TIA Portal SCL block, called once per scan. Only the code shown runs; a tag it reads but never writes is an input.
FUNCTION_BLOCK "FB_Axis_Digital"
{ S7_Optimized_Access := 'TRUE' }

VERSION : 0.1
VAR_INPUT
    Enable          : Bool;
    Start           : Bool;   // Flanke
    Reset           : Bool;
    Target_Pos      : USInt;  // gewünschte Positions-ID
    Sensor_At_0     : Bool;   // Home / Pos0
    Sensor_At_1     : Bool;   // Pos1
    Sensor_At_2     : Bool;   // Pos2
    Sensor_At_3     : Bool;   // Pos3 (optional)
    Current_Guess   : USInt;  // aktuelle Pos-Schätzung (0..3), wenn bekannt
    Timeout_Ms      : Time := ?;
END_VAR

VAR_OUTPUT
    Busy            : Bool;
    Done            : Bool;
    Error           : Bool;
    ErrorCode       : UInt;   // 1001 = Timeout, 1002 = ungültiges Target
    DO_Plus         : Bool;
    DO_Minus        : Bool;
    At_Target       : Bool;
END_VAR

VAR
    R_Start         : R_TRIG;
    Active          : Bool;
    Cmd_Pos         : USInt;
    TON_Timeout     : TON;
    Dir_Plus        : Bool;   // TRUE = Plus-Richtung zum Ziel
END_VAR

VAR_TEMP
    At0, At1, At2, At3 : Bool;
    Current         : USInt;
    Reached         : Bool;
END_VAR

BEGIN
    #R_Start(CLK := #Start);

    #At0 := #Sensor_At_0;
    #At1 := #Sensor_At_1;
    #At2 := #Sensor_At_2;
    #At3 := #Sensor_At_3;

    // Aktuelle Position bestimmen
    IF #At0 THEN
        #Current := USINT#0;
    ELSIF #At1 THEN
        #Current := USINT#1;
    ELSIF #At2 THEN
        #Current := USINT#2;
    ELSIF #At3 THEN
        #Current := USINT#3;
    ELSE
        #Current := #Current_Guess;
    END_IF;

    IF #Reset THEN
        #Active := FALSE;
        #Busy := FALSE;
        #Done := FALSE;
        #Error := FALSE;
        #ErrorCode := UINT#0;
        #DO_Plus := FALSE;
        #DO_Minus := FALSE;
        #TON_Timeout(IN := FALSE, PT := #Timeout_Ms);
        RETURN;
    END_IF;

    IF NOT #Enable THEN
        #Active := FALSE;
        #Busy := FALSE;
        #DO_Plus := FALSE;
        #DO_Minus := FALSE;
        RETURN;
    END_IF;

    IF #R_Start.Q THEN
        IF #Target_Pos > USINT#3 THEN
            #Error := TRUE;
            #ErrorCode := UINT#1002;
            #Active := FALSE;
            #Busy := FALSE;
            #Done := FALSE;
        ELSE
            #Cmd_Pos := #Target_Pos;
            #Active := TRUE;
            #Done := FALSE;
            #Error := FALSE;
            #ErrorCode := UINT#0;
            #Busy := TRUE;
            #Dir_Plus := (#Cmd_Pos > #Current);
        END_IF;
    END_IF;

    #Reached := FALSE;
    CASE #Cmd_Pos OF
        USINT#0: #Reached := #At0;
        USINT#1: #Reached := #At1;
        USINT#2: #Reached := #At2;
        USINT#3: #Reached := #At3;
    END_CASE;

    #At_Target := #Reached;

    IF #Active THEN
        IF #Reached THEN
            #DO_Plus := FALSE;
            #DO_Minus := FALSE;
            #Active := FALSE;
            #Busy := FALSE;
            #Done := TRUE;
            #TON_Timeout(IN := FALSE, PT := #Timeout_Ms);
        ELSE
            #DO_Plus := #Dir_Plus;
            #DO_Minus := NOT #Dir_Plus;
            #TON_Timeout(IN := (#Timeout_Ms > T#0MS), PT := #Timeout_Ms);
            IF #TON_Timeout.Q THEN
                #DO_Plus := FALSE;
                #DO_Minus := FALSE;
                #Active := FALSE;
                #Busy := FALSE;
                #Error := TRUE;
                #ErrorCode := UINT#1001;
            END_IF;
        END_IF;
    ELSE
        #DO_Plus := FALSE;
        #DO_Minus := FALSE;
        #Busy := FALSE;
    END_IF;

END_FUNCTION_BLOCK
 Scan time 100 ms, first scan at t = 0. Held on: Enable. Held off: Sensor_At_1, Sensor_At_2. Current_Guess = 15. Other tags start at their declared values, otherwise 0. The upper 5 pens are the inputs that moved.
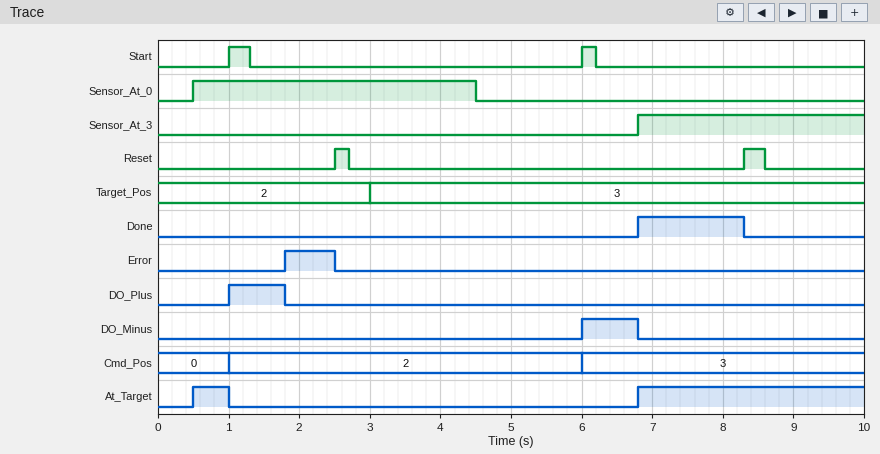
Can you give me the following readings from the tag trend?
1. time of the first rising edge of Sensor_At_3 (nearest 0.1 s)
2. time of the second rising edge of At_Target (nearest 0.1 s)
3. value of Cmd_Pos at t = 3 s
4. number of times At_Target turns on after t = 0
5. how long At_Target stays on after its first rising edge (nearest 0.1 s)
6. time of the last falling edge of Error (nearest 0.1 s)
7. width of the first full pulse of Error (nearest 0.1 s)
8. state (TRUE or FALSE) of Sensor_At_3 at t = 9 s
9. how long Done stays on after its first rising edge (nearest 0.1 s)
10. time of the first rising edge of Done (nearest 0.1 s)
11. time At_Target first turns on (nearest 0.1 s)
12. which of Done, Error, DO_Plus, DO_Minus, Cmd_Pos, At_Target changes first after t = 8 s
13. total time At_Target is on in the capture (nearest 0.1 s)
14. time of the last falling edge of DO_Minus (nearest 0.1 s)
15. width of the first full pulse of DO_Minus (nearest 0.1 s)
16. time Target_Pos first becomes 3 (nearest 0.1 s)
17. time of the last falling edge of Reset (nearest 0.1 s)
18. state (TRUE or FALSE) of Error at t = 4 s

6.8 s
6.8 s
2
2
0.5 s
2.5 s
0.7 s
TRUE
1.5 s
6.8 s
0.5 s
Done
3.7 s
6.8 s
0.8 s
3.0 s
8.6 s
FALSE
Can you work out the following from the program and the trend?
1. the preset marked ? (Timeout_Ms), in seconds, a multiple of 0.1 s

0.8 s
